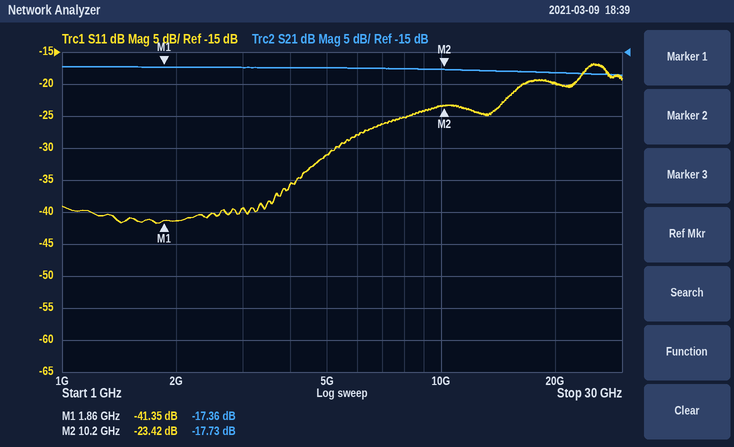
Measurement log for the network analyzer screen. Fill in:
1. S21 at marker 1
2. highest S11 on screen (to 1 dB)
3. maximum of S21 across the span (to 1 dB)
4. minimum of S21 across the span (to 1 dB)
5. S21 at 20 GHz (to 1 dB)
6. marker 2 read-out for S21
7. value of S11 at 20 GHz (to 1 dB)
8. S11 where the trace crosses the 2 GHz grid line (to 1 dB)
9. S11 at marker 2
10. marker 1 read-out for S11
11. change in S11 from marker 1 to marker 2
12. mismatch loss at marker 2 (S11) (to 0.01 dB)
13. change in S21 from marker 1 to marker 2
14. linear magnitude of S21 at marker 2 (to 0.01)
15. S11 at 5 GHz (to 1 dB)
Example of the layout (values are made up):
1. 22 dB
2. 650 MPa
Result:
1. -17.36 dB
2. -17 dB
3. -17 dB
4. -19 dB
5. -18 dB
6. -17.73 dB
7. -20 dB
8. -41 dB
9. -23.42 dB
10. -41.35 dB
11. 17.93 dB
12. 0.02 dB
13. -0.37 dB
14. 0.13
15. -31 dB
